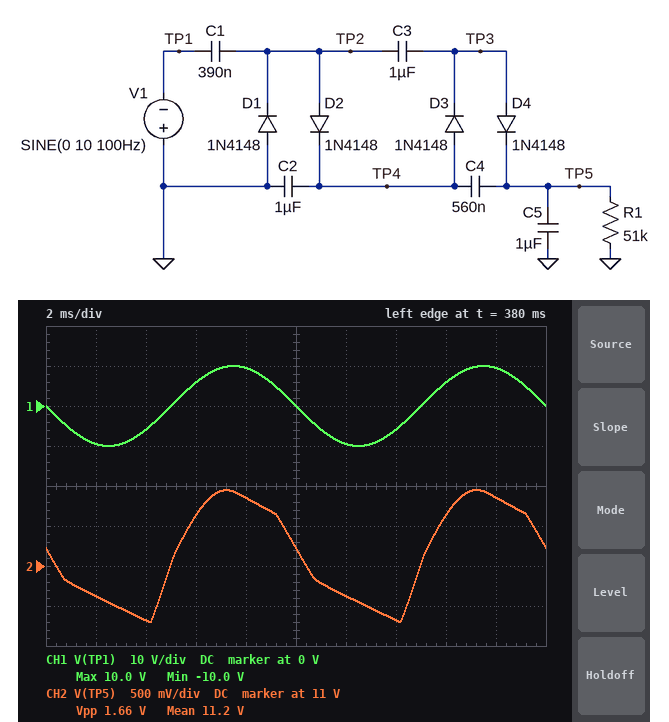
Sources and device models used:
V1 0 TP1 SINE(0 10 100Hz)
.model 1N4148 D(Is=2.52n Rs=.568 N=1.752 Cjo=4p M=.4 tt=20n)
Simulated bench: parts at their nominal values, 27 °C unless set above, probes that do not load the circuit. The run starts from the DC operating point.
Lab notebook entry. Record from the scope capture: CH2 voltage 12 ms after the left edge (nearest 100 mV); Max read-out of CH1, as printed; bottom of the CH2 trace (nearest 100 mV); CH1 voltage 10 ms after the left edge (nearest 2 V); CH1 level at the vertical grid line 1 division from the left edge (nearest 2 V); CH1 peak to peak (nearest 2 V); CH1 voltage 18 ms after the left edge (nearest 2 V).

10.6 V
10.0 V
10.3 V
0 V
-10 V
20 V
10 V
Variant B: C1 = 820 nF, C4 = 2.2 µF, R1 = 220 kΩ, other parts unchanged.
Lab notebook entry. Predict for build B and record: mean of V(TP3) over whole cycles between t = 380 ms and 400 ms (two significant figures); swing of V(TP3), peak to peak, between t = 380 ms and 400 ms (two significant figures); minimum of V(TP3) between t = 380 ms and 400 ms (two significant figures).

21 V
15 V
14 V
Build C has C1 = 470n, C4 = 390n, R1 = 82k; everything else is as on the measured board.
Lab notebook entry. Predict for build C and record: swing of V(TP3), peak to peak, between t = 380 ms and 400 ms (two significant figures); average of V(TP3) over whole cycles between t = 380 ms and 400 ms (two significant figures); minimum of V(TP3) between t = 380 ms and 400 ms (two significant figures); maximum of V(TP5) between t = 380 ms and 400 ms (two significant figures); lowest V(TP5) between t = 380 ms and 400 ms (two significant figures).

9.6 V
13 V
8.2 V
17 V
16 V
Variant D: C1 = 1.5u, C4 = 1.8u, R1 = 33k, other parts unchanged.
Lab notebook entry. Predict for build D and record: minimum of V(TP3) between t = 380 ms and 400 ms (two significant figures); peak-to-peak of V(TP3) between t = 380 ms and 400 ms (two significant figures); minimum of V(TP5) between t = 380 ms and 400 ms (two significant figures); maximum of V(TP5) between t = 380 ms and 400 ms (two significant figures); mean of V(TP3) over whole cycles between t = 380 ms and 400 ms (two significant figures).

8.6 V
9.3 V
14 V
17 V
13 V
